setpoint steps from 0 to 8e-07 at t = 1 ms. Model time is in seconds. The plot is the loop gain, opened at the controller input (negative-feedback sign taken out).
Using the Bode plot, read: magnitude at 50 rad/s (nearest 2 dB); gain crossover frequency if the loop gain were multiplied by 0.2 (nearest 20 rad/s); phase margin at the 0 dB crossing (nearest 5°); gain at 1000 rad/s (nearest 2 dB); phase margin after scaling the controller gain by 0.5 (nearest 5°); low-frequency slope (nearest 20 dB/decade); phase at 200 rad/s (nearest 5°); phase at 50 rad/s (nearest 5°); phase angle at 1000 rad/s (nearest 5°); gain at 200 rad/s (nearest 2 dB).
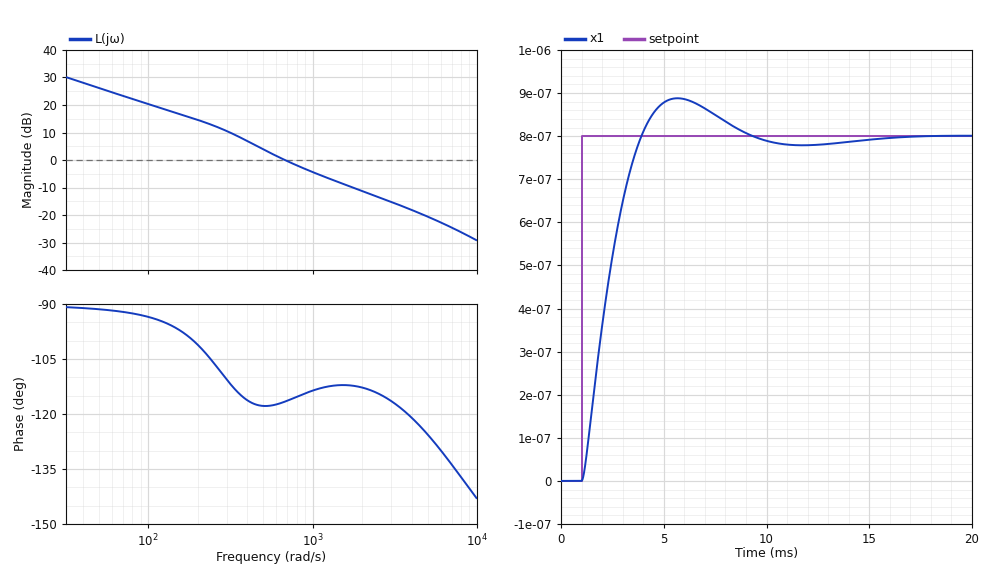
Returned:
26 dB
220 rad/s
65°
-4 dB
65°
-20 dB/decade
-100°
-90°
-115°
14 dB
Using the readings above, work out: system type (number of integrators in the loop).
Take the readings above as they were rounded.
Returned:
1
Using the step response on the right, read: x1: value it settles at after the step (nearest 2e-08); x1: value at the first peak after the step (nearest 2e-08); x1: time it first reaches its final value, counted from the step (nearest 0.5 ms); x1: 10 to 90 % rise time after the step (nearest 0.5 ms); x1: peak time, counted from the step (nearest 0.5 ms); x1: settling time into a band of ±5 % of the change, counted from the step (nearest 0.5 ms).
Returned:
0.00000080
0.00000088
3.0 ms
2.0 ms
4.5 ms
7.0 ms
